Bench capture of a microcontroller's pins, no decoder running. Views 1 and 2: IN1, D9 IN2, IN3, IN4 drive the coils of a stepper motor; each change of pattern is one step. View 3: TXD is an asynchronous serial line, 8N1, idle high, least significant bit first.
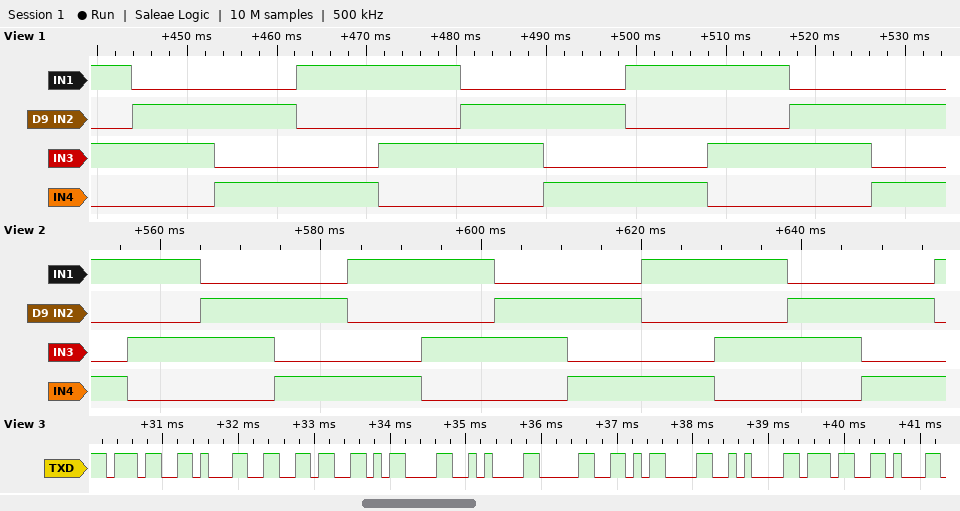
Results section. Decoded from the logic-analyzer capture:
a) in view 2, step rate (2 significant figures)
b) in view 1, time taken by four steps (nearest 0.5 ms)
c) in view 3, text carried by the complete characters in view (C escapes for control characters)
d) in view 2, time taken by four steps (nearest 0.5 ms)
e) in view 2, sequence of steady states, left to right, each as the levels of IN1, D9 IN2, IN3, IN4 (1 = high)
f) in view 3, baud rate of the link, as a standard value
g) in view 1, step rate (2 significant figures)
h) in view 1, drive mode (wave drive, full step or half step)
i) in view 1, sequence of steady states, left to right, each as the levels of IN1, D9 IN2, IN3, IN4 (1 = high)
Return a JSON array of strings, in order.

["110 steps/s", "36.5 ms", "\"716\\r\\n0\\r\\n7\"", "36.5 ms", "1001 1010 0110 0101 1001 1010 0110 0101 1001 1010 0110 0101 1001", "9600 baud", "110 steps/s", "full step", "1010 0110 0101 1001 1010 0110 0101 1001 1010 0110 0101"]
